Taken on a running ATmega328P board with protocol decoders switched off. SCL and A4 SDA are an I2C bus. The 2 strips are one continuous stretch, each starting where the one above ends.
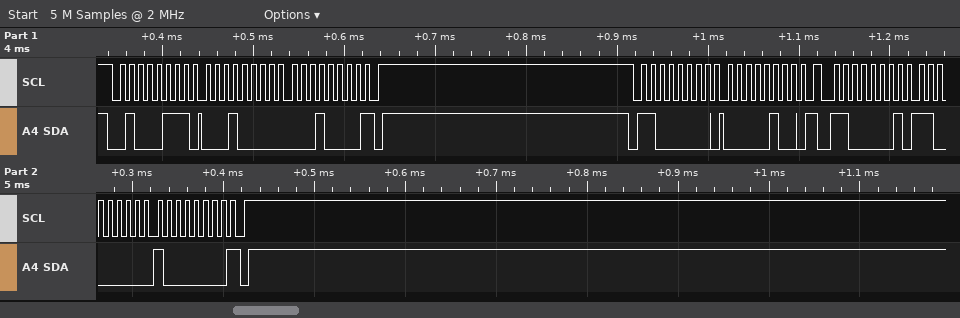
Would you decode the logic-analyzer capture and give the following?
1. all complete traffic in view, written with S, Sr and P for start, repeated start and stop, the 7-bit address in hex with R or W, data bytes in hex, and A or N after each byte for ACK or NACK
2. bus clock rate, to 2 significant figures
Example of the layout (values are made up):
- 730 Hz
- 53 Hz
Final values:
- S 23R A 10 A 10 N P S 60W A 04 A Sr 60R A C0 A 80 N P
- 100 kHz
